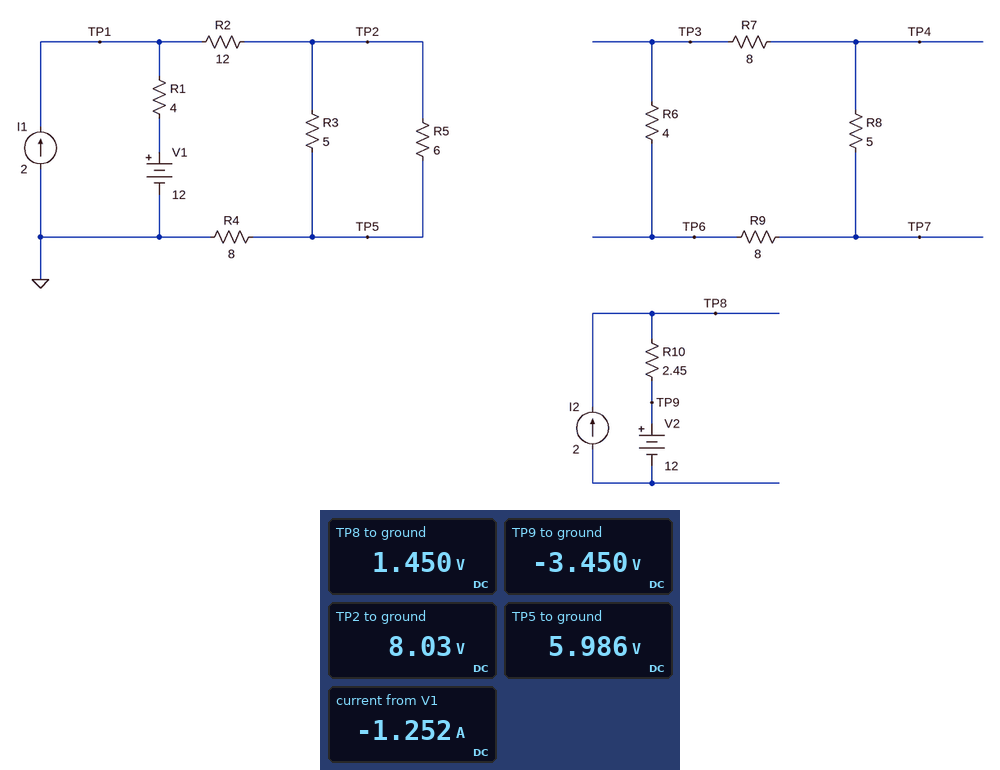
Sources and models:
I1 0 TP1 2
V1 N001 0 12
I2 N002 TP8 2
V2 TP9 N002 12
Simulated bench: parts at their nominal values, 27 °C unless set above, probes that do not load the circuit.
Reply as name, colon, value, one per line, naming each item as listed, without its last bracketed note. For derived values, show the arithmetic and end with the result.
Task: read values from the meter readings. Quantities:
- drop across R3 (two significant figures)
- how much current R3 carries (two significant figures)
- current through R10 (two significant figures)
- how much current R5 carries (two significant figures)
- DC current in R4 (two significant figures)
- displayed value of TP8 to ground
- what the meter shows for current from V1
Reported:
drop across R3: 8.03 V - 5.986 V = 2.0 V
how much current R3 carries: (8.03 V - 5.986 V) / 5 Ω = 410 mA
current through R10: (1.45 V - (-3.45 V)) / 2.45 Ω = 2.0 A
how much current R5 carries: (8.03 V - 5.986 V) / 6 Ω = 340 mA
DC current in R4: (5.986 V) / 8 Ω = 750 mA
displayed value of TP8 to ground: 1.450 V
what the meter shows for current from V1: -1.252 A
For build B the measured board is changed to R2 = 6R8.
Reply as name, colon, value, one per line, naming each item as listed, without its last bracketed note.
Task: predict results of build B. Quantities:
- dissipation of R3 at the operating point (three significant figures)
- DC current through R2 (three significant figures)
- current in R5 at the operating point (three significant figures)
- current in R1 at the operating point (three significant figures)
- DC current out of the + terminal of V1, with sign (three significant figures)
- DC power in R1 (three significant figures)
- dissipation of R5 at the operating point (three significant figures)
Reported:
dissipation of R3 at the operating point: 1.28 W
DC current through R2: 929 mA
current in R5 at the operating point: 422 mA
current in R1 at the operating point: 1.07 A
DC current out of the + terminal of V1, with sign: -1.07 A
DC power in R1: 4.59 W
dissipation of R5 at the operating point: 1.07 W
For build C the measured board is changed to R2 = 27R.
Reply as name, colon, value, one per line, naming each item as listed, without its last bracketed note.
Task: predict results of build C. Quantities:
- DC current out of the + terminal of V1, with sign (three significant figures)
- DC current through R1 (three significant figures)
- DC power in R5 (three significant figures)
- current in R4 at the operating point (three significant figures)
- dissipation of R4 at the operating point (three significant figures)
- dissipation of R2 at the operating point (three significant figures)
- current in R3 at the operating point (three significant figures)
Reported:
DC current out of the + terminal of V1, with sign: -1.52 A
DC current through R1: 1.52 A
DC power in R5: 285 mW
current in R4 at the operating point: 479 mA
dissipation of R4 at the operating point: 1.84 W
dissipation of R2 at the operating point: 6.20 W
current in R3 at the operating point: 261 mA
